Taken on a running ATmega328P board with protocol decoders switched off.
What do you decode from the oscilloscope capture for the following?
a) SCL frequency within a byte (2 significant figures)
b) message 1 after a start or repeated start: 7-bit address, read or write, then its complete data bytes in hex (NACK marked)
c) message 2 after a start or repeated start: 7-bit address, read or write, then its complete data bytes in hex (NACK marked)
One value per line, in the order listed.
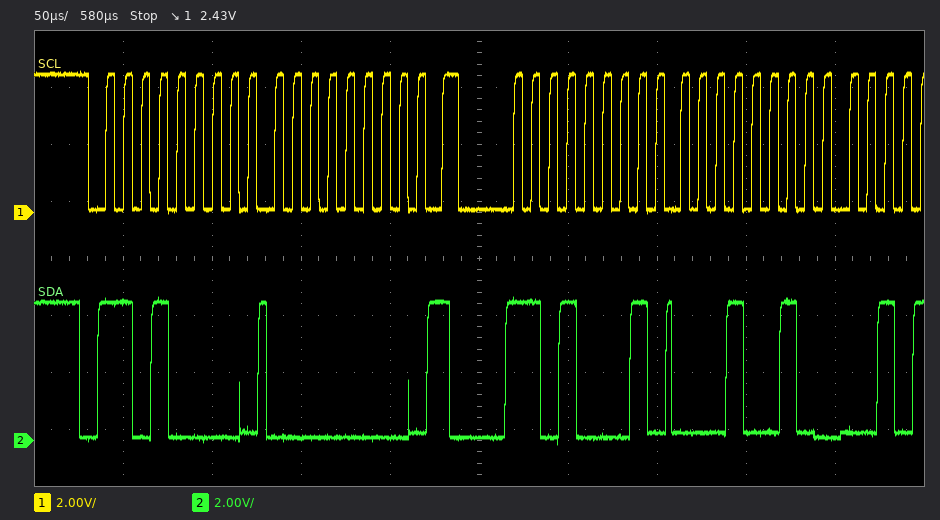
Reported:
100 kHz
0x68 write: 00
0x68 read: 12
